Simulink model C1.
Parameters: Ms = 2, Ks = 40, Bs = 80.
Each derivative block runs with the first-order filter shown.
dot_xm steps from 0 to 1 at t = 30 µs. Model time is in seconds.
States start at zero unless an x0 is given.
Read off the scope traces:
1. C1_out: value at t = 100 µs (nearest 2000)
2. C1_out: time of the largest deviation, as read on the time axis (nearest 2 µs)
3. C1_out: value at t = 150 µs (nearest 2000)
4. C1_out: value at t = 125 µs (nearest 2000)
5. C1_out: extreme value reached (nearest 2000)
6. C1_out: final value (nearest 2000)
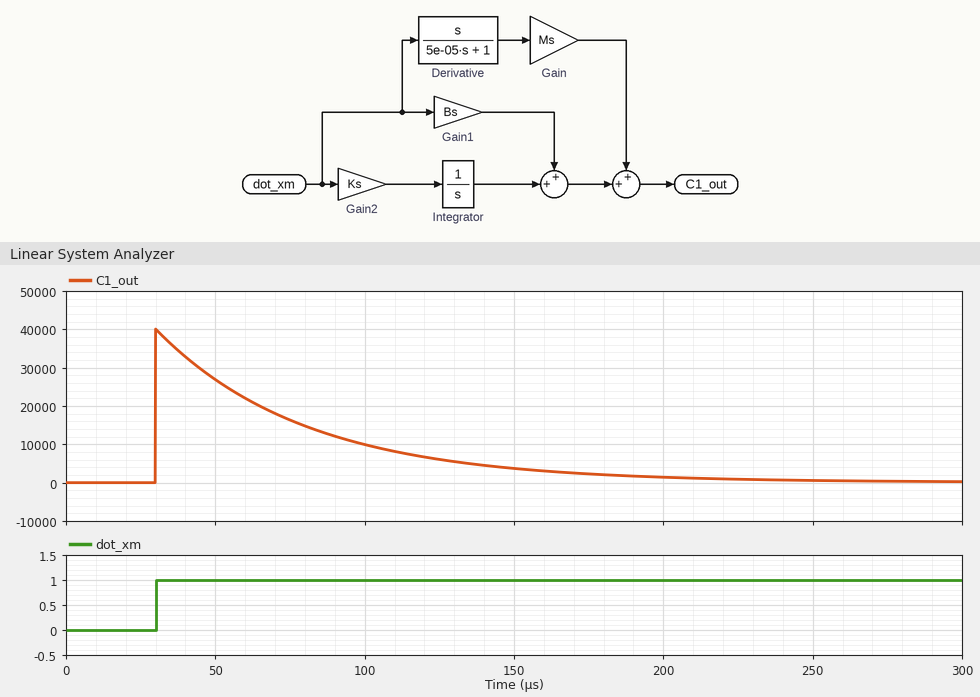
10000
30 µs
4000
6000
40000
0
